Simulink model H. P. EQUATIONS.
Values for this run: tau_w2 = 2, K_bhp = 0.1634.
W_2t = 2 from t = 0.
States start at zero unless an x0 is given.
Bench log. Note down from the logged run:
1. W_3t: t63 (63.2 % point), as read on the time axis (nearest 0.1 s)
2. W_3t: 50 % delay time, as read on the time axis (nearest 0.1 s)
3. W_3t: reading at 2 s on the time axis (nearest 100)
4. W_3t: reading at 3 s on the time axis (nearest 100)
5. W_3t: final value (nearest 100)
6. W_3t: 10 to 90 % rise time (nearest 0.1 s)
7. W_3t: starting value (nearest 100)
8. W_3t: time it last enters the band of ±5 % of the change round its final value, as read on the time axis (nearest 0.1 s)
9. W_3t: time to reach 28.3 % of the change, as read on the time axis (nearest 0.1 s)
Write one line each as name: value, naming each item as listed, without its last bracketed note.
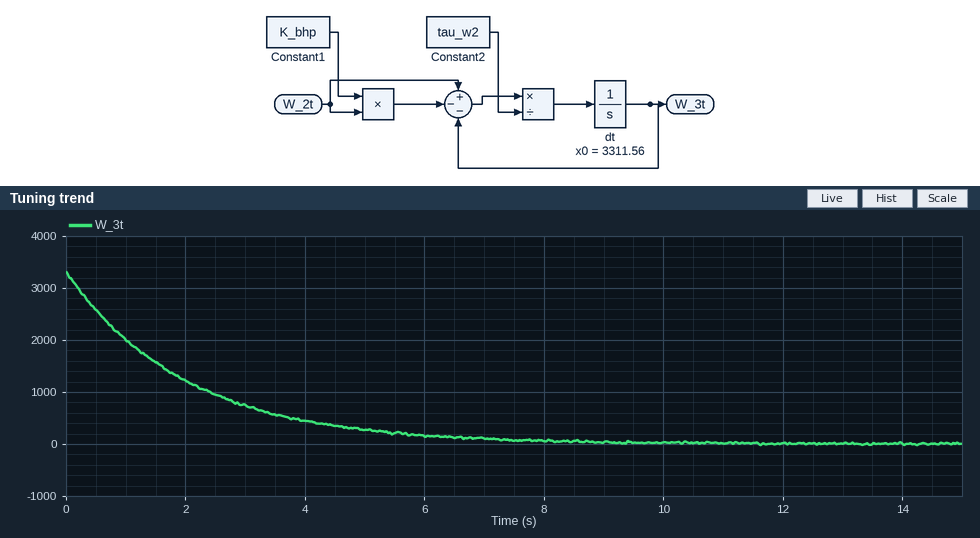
W_3t: t63 (63.2 % point), as read on the time axis: 2.0 s
W_3t: 50 % delay time, as read on the time axis: 1.4 s
W_3t: reading at 2 s on the time axis: 1200
W_3t: reading at 3 s on the time axis: 700
W_3t: final value: 0
W_3t: 10 to 90 % rise time: 4.4 s
W_3t: starting value: 3300
W_3t: time it last enters the band of ±5 % of the change round its final value, as read on the time axis: 6.0 s
W_3t: time to reach 28.3 % of the change, as read on the time axis: 0.7 s
